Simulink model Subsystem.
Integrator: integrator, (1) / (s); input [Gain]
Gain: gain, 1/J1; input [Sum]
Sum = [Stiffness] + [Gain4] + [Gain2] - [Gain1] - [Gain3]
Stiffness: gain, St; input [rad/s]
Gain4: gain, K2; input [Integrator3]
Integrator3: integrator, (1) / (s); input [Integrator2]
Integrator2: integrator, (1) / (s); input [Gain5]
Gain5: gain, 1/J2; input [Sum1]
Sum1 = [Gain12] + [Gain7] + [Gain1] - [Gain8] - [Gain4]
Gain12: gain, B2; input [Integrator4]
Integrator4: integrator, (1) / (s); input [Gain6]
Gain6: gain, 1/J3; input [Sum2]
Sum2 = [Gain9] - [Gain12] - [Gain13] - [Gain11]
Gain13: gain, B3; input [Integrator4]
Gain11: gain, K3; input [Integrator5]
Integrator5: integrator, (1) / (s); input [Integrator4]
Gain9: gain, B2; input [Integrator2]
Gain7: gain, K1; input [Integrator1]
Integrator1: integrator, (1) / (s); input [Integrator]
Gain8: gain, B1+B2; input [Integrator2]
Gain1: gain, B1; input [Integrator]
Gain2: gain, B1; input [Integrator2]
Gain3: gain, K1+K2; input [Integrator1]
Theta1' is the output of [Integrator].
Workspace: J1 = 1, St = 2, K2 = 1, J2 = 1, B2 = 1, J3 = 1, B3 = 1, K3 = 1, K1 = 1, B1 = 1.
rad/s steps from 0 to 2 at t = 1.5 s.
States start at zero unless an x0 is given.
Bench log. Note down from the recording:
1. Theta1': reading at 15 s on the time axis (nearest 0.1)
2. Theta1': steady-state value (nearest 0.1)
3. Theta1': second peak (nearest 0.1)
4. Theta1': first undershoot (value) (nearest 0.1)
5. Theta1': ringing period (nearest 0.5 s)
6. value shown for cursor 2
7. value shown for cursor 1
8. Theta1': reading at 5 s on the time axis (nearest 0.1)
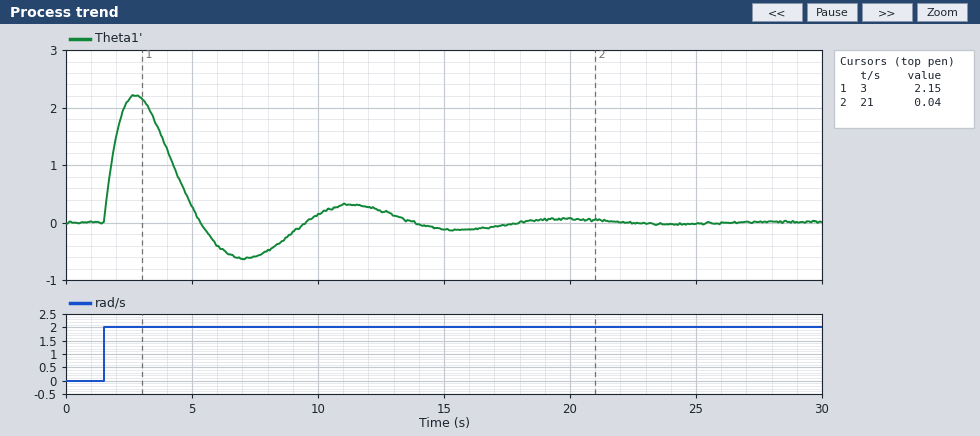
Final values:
-0.1
0.0
0.3
-0.6
8.5 s
0.04
2.15
0.3
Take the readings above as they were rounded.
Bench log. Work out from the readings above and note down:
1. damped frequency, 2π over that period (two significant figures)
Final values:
0.74 rad/s
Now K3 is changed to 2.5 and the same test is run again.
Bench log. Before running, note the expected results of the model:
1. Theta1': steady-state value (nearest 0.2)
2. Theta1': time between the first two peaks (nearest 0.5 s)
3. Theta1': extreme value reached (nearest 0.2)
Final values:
0.0
7.5 s
2.2
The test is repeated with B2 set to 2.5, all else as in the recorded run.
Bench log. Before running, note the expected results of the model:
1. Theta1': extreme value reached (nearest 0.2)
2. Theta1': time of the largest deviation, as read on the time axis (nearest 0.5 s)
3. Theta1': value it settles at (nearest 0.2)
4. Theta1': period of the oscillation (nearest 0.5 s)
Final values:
2.2
2.5 s
0.0
8.0 s
